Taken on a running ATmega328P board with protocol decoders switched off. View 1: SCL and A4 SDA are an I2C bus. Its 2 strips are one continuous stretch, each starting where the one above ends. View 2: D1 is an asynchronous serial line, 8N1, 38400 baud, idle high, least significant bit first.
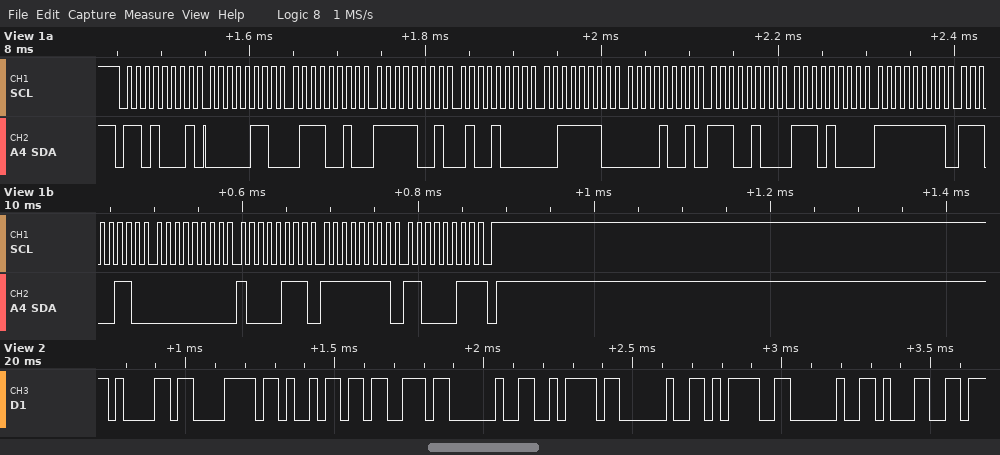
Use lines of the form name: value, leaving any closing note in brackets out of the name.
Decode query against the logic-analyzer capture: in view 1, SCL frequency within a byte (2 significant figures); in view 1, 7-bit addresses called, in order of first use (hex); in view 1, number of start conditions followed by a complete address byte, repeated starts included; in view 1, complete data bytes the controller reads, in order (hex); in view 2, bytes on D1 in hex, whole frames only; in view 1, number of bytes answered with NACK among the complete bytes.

in view 1, SCL frequency within a byte: 100 kHz
in view 1, 7-bit addresses called, in order of first use: 0x68
in view 1, number of start conditions followed by a complete address byte, repeated starts included: 1
in view 1, complete data bytes the controller reads, in order: 06 72 F9 48 3E 09 E4 E8 FF E6 00 87 FF C3
in view 2, bytes on D1 in hex, whole frames only: 0x61 0x78 0x69 0x73 0x20 0x7A 0x20 0x3D 0x20 0x31
in view 1, number of bytes answered with NACK among the complete bytes: 1
